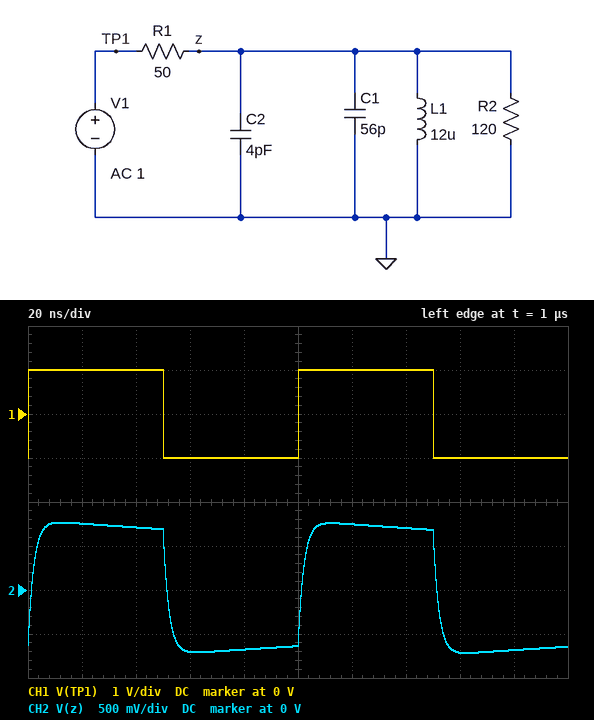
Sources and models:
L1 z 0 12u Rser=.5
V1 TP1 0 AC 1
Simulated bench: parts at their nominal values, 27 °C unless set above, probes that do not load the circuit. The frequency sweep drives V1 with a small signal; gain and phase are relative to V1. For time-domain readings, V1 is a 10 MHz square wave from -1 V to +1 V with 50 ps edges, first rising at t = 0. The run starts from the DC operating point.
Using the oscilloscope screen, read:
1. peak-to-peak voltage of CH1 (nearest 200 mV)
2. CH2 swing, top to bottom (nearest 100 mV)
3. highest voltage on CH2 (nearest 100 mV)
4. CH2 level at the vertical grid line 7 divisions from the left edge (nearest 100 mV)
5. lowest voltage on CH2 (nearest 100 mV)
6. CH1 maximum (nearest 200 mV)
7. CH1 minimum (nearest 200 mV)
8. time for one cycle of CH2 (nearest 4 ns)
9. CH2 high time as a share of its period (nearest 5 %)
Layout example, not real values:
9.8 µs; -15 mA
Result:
2.0 V; 1.5 V; 800 mV; 700 mV; -700 mV; 1.0 V; -1.0 V; 100 ns; 50 %
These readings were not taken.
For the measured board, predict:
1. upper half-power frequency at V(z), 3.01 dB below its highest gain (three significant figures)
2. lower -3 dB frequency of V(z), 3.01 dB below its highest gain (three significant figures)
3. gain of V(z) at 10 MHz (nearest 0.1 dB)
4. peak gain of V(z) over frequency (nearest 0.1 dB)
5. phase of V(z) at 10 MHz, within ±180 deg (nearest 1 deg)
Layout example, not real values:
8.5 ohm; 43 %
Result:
75.6 MHz; 472 kHz; -3.1 dB; -3.0 dB; -5 deg
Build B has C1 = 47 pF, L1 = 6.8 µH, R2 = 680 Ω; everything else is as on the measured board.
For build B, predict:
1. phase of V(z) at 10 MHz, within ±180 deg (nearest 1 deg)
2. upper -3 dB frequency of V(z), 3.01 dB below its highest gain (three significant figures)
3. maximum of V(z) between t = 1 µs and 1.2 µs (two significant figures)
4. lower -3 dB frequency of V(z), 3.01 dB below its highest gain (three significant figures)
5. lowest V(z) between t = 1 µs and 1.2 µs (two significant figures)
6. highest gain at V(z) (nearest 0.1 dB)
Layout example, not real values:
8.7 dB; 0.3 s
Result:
-2 deg; 68.1 MHz; 1.0 V; 1.08 MHz; -1.0 V; -0.6 dB
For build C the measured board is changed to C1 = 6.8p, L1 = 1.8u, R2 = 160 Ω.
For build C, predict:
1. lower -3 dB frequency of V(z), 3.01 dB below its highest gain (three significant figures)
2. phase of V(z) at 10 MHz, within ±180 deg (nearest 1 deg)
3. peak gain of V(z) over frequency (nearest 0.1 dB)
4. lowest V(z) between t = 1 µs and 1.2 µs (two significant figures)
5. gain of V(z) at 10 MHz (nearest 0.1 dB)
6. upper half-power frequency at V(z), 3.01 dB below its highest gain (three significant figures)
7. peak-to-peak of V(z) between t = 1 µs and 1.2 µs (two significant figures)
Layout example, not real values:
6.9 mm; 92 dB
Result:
3.38 MHz; 17 deg; -2.4 dB; -1.1 V; -2.8 dB; 390 MHz; 2.2 V
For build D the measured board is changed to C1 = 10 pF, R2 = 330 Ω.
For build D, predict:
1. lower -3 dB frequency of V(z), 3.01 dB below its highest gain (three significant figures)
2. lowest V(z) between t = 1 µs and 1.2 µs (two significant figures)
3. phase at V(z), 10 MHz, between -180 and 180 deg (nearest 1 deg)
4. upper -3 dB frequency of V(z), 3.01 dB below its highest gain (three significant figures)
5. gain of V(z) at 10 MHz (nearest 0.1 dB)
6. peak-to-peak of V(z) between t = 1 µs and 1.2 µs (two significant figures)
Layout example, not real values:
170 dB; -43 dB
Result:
581 kHz; -920 mV; 1 deg; 262 MHz; -1.2 dB; 1.9 V
